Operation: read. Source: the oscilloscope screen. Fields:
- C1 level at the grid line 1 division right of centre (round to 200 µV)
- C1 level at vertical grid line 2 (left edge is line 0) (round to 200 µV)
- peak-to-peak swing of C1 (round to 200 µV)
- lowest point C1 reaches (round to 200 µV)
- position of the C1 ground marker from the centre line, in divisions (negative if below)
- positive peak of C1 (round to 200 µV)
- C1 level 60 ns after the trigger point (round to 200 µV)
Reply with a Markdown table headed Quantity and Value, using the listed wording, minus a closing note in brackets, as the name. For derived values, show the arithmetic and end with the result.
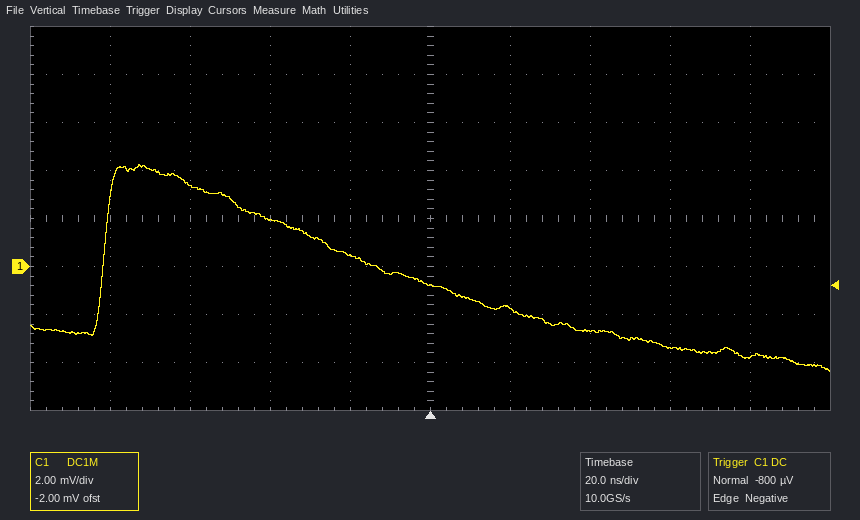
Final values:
| Quantity | Value |
|---|---|
| C1 level at the grid line 1 division right of centre | -1.8 mV |
| C1 level at vertical grid line 2 (left edge is line 0) | 3.4 mV |
| peak-to-peak swing of C1 | 4.2 mV − (-4.4 mV) = 8.6 mV |
| lowest point C1 reaches | -4.4 mV |
| position of the C1 ground marker from the centre line, in divisions | -1.0 div |
| positive peak of C1 | 4.2 mV |
| C1 level 60 ns after the trigger point | -3.4 mV |
